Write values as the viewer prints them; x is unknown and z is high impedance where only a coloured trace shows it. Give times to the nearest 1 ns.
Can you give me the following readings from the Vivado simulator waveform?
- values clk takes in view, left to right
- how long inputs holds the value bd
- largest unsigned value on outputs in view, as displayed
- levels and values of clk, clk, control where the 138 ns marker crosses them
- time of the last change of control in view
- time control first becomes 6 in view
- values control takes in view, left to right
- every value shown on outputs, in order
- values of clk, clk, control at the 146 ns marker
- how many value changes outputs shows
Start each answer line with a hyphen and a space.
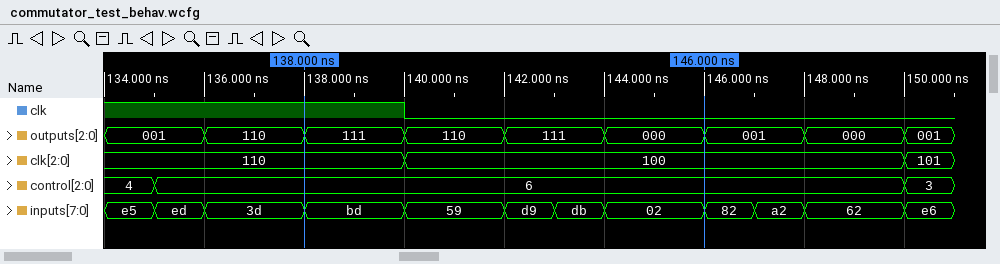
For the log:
- 110, 100, 101
- 2 ns
- 111
- clk=110, clk=110, control=6
- 150 ns
- 135 ns
- 4, 6, 3
- 001, 110, 111, 110, 111, 000, 001, 000, 001
- clk=100, clk=100, control=6
- 8
